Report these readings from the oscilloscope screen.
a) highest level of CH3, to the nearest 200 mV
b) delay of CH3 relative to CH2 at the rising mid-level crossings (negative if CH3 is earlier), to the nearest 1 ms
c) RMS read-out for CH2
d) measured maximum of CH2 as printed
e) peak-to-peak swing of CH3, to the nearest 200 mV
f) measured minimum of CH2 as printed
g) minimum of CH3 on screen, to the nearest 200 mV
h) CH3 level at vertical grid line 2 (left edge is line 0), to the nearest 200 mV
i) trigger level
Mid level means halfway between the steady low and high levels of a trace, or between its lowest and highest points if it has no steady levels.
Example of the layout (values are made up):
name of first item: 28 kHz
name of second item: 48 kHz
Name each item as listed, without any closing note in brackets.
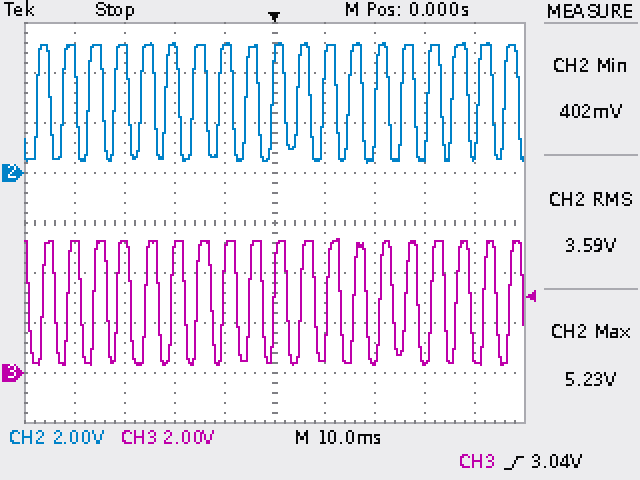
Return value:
highest level of CH3, to the nearest 200 mV: 5.4 V
delay of CH3 relative to CH2 at the rising mid-level crossings (negative if CH3 is earlier), to the nearest 1 ms: +1 ms
RMS read-out for CH2: 3.59 V
measured maximum of CH2 as printed: 5.23 V
peak-to-peak swing of CH3, to the nearest 200 mV: 5.0 V
measured minimum of CH2 as printed: 402 mV
minimum of CH3 on screen, to the nearest 200 mV: 400 mV
CH3 level at vertical grid line 2 (left edge is line 0), to the nearest 200 mV: 5.2 V
trigger level: 3.04 V
